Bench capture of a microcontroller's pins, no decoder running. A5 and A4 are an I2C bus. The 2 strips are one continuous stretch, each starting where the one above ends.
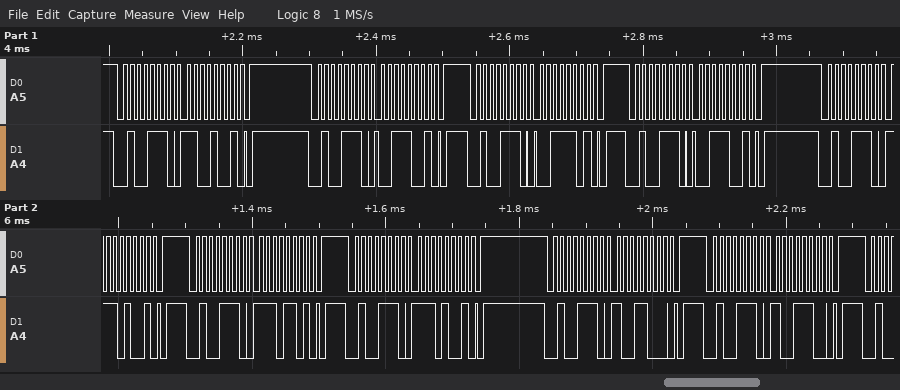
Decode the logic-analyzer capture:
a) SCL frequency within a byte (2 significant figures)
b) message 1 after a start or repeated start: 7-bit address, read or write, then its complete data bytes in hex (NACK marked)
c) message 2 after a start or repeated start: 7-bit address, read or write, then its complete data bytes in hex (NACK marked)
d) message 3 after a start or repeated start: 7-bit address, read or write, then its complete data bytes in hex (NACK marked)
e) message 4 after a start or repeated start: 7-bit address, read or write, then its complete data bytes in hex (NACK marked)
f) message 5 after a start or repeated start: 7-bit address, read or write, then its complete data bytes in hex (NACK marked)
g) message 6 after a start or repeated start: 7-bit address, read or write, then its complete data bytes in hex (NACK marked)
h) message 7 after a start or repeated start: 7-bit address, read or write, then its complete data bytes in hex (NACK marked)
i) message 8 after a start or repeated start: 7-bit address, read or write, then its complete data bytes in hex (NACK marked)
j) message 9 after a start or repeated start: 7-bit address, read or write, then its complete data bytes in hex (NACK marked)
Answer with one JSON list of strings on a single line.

["100 kHz", "0x27 write: C9", "0x27 write: 39", "0x27 write: 3D", "0x27 write: 39", "0x27 write: E9", "0x27 write: ED", "0x27 write: E9", "0x27 write: 98", "0x27 write: 9C"]
